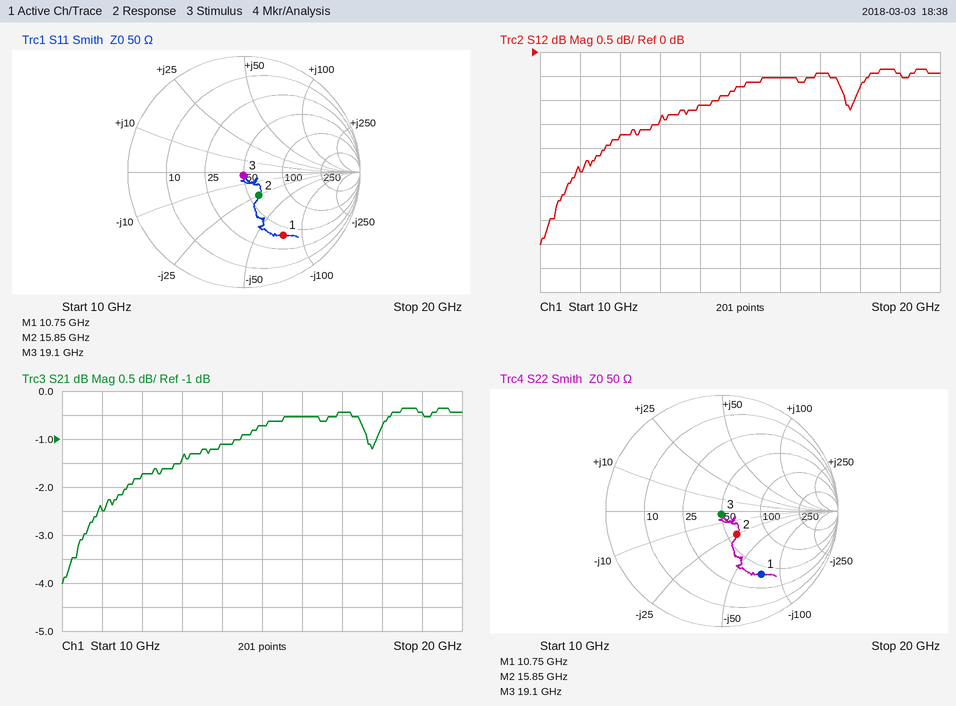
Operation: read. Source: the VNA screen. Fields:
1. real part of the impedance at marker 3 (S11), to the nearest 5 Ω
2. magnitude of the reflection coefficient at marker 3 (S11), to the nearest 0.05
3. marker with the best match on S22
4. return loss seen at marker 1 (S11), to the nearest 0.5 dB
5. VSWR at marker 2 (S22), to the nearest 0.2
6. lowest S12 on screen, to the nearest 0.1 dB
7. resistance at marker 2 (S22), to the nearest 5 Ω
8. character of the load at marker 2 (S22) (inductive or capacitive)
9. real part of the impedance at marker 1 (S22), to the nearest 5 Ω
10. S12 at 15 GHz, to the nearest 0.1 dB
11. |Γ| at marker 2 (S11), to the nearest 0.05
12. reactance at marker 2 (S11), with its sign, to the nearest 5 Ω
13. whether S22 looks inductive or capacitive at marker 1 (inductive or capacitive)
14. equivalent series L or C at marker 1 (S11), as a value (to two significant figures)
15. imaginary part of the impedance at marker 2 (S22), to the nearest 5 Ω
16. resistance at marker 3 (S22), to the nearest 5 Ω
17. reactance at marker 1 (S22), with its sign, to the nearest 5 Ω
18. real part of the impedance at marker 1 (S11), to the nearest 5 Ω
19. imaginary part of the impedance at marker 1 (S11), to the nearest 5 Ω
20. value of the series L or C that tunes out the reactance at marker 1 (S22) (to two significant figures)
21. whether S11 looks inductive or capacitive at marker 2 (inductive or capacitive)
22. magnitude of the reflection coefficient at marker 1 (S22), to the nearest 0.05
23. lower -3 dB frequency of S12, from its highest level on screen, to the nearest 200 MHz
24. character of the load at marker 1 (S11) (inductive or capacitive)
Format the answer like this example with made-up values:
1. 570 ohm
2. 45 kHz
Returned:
1. 50 Ω
2. 0.05
3. marker 3
4. 4.0 dB
5. 1.6
6. -4.0 dB
7. 60 Ω
8. capacitive
9. 40 Ω
10. -0.7 dB
11. 0.25
12. -25 Ω
13. capacitive
14. 200 fF
15. -25 Ω
16. 50 Ω
17. -75 Ω
18. 40 Ω
19. -75 Ω
20. 1.1 nH
21. capacitive
22. 0.65
23. 10.4 GHz
24. capacitive
